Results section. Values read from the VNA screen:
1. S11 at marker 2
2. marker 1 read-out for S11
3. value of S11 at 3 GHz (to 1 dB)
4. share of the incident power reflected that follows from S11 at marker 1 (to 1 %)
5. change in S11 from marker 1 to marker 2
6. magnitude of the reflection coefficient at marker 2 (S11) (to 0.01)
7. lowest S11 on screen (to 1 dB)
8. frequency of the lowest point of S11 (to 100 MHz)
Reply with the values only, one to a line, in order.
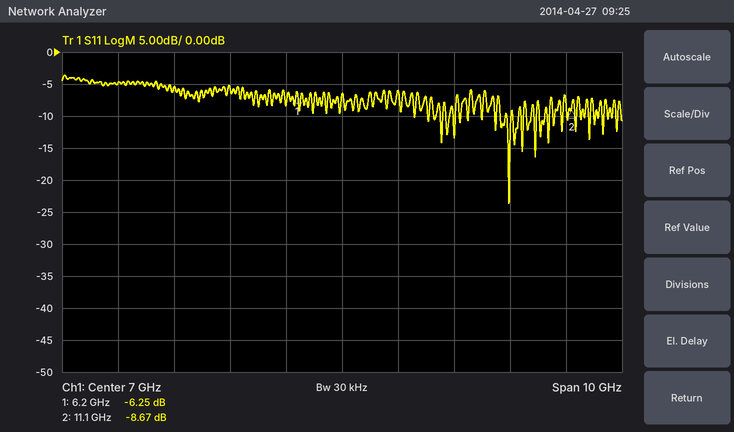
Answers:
-8.67 dB
-6.25 dB
-5 dB
24 %
-2.42 dB
0.37
-24 dB
10.0 GHz
